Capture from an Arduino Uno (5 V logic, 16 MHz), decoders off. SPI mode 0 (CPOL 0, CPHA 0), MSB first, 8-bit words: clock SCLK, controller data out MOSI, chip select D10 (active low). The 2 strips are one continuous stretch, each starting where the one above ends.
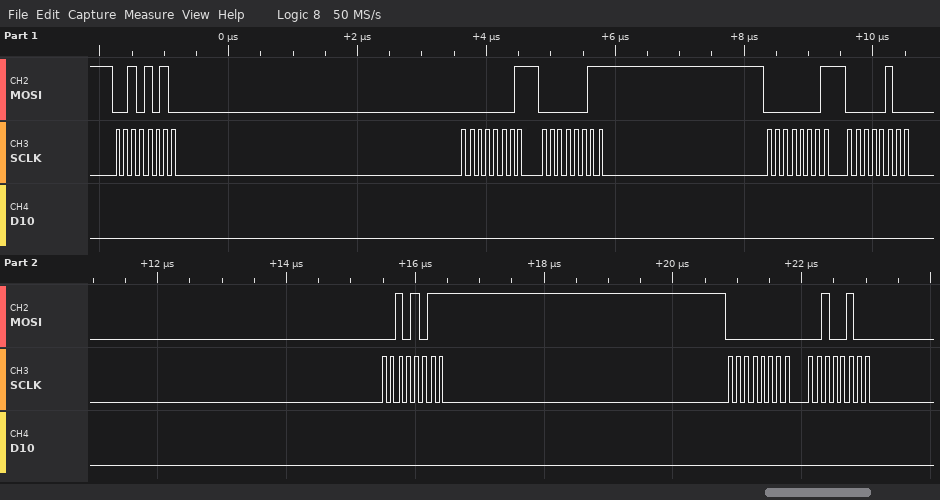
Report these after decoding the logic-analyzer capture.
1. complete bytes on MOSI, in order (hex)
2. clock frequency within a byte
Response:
2A 01 03 01 04 2B 00 24
8 MHz
